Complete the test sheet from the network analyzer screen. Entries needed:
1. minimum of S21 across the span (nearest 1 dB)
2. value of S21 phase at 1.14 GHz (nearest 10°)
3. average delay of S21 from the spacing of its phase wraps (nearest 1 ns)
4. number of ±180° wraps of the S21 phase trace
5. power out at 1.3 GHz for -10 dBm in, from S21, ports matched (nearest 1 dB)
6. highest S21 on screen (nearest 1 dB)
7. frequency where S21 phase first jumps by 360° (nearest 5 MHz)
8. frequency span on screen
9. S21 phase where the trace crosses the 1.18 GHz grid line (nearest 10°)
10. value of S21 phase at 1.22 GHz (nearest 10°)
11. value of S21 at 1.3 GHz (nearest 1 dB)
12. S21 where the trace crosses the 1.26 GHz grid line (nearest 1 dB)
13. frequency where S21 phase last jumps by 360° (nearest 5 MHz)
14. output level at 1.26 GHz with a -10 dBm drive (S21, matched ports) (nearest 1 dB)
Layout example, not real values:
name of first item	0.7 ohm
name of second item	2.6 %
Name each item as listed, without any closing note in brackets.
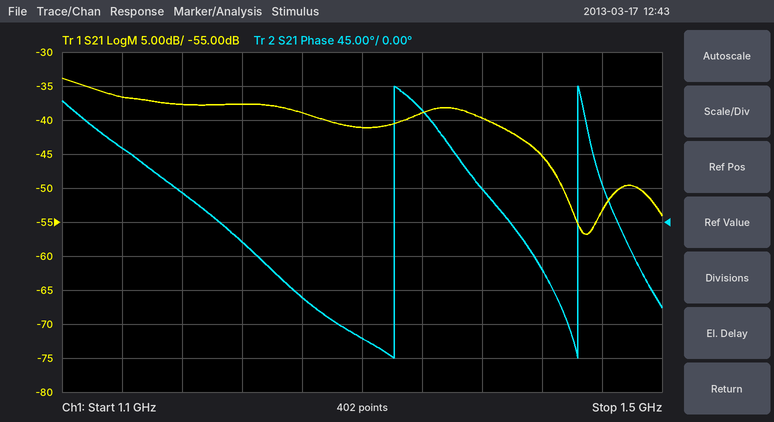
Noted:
minimum of S21 across the span	-57 dB
value of S21 phase at 1.14 GHz	100°
average delay of S21 from the spacing of its phase wraps	8 ns
number of ±180° wraps of the S21 phase trace	2
power out at 1.3 GHz for -10 dBm in, from S21, ports matched	-51 dBm
highest S21 on screen	-34 dB
frequency where S21 phase first jumps by 360°	1.320 GHz
frequency span on screen	400 MHz
S21 phase where the trace crosses the 1.18 GHz grid line	40°
value of S21 phase at 1.22 GHz	-30°
value of S21 at 1.3 GHz	-41 dB
S21 where the trace crosses the 1.26 GHz grid line	-39 dB
frequency where S21 phase last jumps by 360°	1.445 GHz
output level at 1.26 GHz with a -10 dBm drive (S21, matched ports)	-49 dBm
